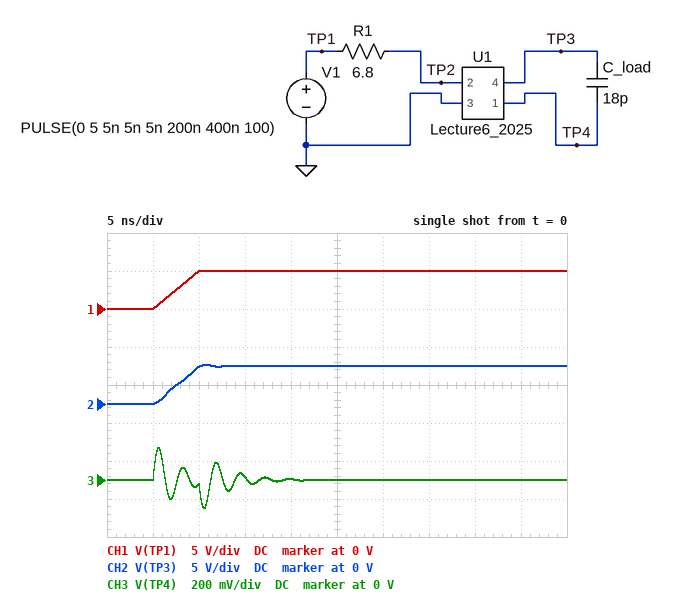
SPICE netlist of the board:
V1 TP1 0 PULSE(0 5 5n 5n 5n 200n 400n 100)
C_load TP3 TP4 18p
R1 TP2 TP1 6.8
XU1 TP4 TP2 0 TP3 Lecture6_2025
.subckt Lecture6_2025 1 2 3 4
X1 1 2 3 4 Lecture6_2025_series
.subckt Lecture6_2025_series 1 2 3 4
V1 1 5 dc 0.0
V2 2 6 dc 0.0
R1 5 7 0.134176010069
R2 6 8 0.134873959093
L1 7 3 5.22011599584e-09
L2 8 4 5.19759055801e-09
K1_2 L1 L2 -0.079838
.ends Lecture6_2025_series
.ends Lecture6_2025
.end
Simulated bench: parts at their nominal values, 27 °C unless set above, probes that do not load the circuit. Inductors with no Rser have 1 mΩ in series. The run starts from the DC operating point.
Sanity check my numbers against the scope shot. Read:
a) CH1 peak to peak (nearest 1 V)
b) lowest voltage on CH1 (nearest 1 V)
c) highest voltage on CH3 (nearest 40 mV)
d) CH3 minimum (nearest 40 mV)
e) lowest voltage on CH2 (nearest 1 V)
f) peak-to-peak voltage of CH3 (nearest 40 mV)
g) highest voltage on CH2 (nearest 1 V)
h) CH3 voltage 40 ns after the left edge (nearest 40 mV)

5 V
0 V
160 mV
-160 mV
0 V
320 mV
5 V
0 V
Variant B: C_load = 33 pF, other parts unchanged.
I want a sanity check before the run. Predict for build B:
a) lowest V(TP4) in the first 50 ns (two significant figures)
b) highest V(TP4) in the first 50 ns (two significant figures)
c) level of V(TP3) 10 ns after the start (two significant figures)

-230 mV
210 mV
4.7 V
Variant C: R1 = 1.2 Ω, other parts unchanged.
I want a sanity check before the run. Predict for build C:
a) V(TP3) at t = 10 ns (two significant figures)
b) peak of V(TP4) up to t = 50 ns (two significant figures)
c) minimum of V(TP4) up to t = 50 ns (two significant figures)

5.1 V
200 mV
-180 mV
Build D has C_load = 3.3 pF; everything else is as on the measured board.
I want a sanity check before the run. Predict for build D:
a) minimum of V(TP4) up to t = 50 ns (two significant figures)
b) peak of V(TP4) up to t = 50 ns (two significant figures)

-93 mV
81 mV
